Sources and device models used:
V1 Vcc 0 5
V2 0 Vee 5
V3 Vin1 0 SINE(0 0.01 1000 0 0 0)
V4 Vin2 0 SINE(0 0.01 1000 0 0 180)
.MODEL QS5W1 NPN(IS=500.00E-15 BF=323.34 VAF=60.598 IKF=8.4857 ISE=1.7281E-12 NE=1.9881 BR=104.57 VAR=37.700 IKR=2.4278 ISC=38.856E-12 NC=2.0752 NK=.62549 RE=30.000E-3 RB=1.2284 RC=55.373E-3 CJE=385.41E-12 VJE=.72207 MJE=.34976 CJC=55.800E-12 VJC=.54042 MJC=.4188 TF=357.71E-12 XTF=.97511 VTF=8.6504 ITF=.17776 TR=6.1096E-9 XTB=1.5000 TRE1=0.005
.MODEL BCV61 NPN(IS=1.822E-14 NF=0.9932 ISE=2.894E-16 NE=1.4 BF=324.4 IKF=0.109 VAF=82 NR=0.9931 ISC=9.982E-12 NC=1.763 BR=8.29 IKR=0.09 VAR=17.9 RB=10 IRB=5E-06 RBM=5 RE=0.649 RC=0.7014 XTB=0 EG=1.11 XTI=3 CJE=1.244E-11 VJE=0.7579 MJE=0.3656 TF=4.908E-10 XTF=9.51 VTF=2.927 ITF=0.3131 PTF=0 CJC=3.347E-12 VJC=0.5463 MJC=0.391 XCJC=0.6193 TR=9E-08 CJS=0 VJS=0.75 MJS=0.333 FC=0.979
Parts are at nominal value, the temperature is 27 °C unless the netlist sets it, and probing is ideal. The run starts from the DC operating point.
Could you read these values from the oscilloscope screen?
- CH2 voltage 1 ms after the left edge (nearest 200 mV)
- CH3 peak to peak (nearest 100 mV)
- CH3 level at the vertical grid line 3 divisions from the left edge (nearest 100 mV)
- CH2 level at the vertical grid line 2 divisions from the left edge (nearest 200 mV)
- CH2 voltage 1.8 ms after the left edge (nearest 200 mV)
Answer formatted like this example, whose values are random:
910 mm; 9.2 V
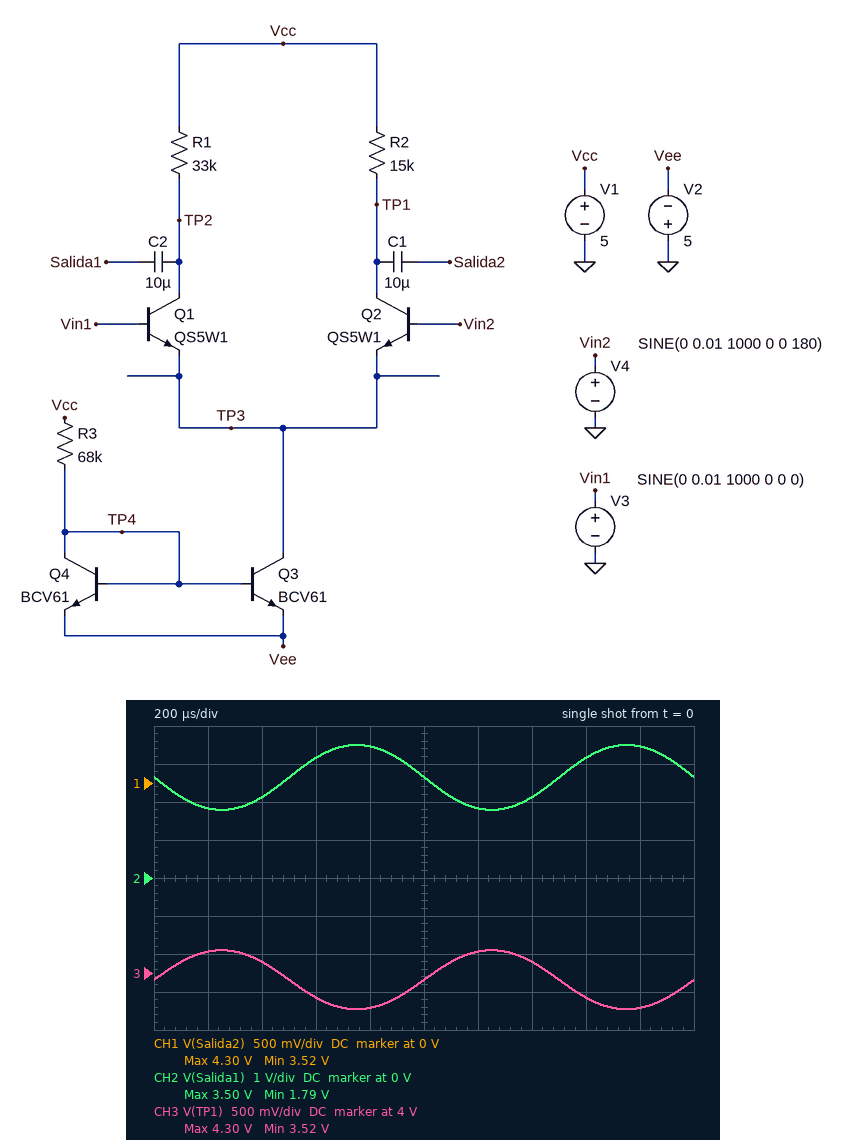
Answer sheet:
2.6 V; 800 mV; 3.7 V; 2.2 V; 3.4 V
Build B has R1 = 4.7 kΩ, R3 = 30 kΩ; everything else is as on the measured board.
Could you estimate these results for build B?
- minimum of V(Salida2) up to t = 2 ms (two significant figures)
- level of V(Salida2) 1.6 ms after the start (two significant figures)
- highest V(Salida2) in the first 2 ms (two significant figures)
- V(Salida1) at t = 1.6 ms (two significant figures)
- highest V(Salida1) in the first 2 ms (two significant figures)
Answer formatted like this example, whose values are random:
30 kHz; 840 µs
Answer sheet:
1.7 V; 2.1 V; 3.5 V; 4.4 V; 4.5 V
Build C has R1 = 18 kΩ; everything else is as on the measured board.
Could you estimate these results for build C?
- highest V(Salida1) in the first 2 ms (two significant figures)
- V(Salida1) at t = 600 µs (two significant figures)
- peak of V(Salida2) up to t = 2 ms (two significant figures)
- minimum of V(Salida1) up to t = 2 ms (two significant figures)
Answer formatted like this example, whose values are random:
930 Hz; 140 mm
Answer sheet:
4.2 V; 4.0 V; 4.3 V; 3.2 V
